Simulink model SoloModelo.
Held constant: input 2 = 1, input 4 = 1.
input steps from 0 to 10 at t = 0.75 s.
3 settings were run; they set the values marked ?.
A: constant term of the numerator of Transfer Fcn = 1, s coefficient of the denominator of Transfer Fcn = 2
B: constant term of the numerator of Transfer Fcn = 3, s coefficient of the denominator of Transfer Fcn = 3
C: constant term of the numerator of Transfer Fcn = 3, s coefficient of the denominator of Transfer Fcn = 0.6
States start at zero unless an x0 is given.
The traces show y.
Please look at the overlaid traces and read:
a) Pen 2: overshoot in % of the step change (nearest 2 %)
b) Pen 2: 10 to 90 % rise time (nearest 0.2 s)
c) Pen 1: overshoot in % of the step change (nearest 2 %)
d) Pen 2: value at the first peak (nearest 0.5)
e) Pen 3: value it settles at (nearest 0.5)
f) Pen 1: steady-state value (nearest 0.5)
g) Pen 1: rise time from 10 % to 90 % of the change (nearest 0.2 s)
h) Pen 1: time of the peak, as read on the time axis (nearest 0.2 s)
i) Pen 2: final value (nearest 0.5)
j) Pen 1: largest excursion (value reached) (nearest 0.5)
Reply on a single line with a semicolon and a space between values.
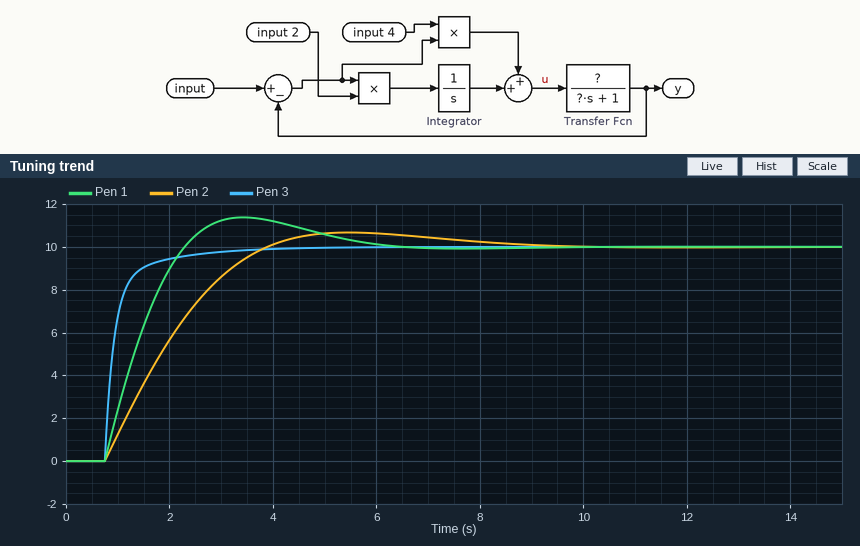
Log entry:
6 %; 2.2 s; 14 %; 10.5; 10.0; 10.0; 1.2 s; 3.4 s; 10.0; 11.5
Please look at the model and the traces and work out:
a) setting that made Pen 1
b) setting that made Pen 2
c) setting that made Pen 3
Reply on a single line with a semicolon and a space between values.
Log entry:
B; A; C
